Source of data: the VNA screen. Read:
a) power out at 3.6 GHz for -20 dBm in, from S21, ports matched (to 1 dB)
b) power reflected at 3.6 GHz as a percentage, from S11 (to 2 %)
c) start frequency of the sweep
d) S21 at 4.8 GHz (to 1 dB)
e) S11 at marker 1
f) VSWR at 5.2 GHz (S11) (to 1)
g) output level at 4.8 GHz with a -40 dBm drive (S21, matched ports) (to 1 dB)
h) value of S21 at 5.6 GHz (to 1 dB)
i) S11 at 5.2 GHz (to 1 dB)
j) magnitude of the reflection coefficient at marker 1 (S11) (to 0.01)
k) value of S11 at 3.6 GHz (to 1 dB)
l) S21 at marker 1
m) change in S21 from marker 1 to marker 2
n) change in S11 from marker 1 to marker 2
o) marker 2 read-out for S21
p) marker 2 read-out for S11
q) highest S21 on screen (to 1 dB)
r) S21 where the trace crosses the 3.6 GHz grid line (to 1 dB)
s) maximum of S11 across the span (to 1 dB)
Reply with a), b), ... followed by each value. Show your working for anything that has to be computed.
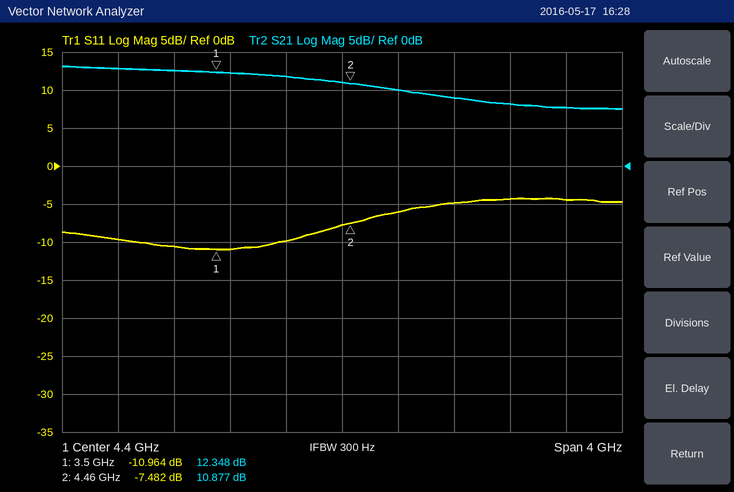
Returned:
a) -20 dBm + (12 dB) = -8 dBm
b) 10^(-11/10) ≈ 8 %
c) 2.4 GHz
d) 10 dB
e) -10.964 dB
f) |Γ| = 10^(-5/20) = 0.5623; VSWR = (1 + 0.5623)/(1 − 0.5623) ≈ 4
g) -40 dBm + (10 dB) = -30 dBm
h) 8 dB
i) -5 dB
j) 10^(-10.964/20) ≈ 0.28
k) -11 dB
l) 12.348 dB
m) 10.877 − (12.348) = -1.471 dB
n) -7.482 − (-10.964) = 3.482 dB
o) 10.877 dB
p) -7.482 dB
q) 13 dB
r) 12 dB
s) -4 dB
